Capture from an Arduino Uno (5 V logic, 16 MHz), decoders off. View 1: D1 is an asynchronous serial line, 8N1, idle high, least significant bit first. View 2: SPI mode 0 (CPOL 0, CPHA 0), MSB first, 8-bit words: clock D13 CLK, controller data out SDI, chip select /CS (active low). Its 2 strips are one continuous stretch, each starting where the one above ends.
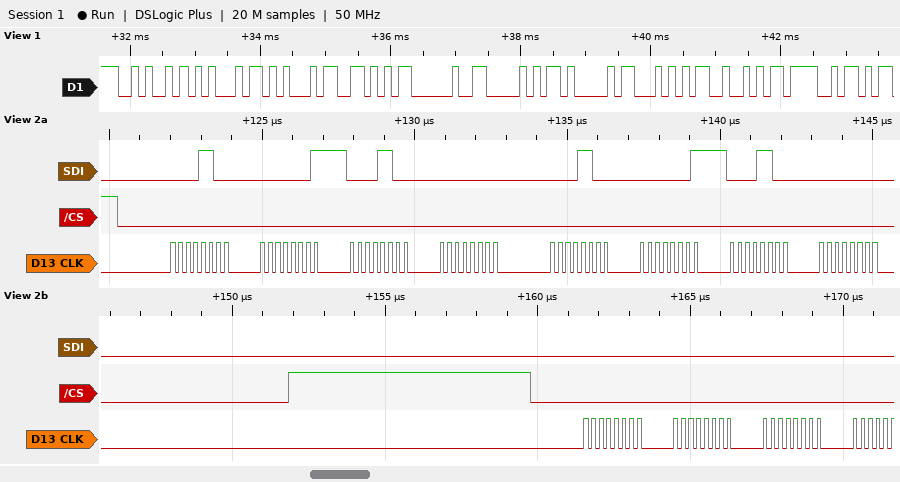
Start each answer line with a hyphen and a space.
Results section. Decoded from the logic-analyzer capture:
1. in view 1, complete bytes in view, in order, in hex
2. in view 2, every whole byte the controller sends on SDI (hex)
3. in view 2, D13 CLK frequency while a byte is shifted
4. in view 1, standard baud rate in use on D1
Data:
- 4A 45 45 56 20 50 41 54 52 4F
- 0C 01 0C 00 0C 01 0C 00 00 00 00
- 4 MHz
- 9600 baud
